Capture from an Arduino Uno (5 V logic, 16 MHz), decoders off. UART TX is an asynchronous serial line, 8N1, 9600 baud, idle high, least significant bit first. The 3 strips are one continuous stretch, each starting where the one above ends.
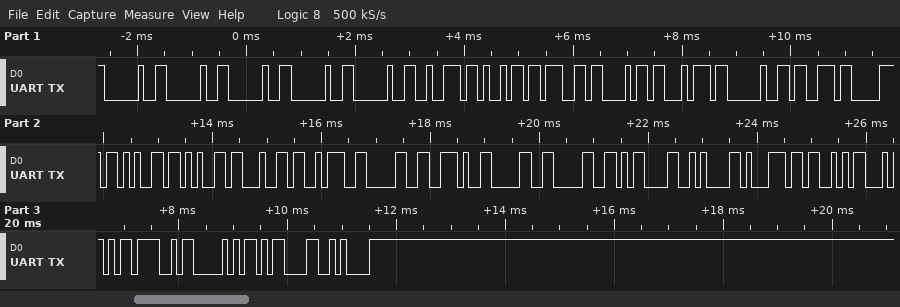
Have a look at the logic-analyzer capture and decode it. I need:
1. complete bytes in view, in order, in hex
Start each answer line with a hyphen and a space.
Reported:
- 20 20 20 20 20 72 69 67 68 74 20 73 70 65 65 64 3A 30 2E 30 30 0D 0A 71 53 54 4F 50 0D 0A
